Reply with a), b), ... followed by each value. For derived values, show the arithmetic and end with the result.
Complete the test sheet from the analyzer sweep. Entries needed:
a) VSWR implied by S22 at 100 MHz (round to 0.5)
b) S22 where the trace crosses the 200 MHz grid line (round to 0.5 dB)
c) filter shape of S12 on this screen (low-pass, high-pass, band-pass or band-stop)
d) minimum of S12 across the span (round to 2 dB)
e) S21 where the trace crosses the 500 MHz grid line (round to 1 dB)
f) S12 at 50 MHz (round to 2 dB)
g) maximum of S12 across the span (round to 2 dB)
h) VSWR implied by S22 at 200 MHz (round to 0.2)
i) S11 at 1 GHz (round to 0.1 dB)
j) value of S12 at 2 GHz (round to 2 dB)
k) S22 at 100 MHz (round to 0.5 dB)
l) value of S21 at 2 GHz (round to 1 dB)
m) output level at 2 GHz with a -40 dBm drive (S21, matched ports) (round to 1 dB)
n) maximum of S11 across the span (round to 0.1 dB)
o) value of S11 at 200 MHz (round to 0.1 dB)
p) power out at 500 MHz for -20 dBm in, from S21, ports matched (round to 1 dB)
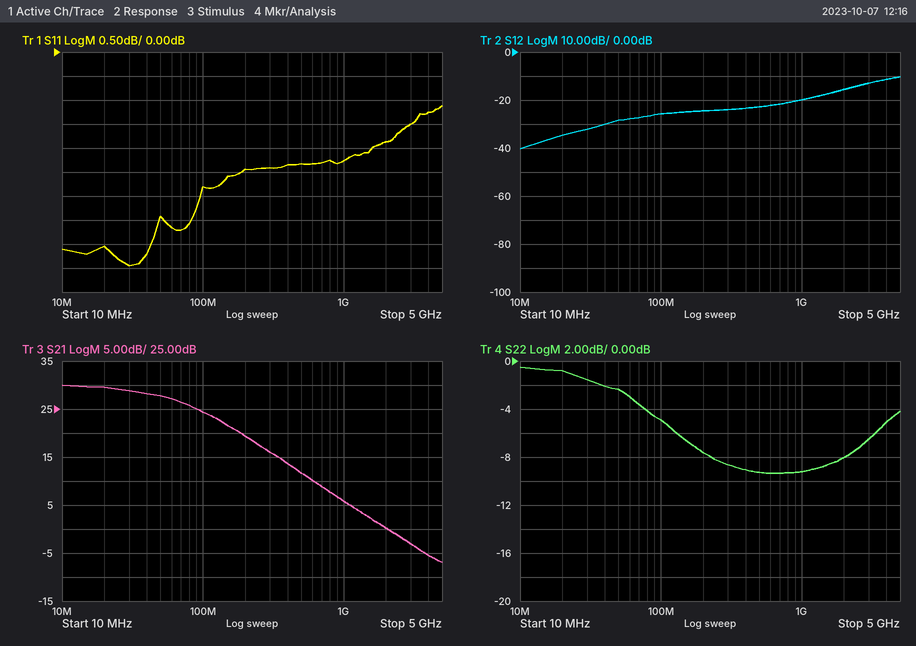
a) |Γ| = 10^(-5/20) = 0.5623; VSWR = (1 + 0.5623)/(1 − 0.5623) ≈ 3.57, so 3.5 to the nearest 0.5
b) -7.5 dB
c) high-pass
d) -40 dB
e) 12 dB
f) -28 dB
g) -10 dB
h) |Γ| = 10^(-7.5/20) = 0.4217; VSWR = (1 + 0.4217)/(1 − 0.4217) ≈ 2.46, so 2.4 to the nearest 0.2
i) -2.3 dB
j) -16 dB
k) -5.0 dB
l) 0 dB
m) -40 dBm + (0 dB) = -40 dBm
n) -1.1 dB
o) -2.4 dB
p) -20 dBm + (12 dB) = -8 dBm
